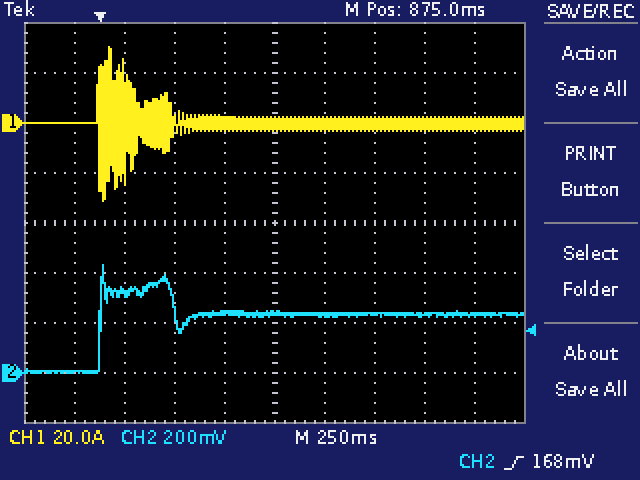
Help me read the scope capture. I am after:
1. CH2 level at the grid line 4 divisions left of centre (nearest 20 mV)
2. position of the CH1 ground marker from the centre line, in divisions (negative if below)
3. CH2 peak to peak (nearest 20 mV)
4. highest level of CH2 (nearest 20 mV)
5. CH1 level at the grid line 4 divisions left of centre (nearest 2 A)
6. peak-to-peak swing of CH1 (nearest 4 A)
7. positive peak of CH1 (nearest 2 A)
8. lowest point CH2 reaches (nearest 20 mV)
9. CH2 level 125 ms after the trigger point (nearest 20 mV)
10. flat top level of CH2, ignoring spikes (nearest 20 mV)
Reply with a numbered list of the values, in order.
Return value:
1. 0 mV
2. +2.0 div
3. 440 mV
4. 440 mV
5. 0 A
6. 60 A
7. 30 A
8. 0 mV
9. 320 mV
10. 240 mV
